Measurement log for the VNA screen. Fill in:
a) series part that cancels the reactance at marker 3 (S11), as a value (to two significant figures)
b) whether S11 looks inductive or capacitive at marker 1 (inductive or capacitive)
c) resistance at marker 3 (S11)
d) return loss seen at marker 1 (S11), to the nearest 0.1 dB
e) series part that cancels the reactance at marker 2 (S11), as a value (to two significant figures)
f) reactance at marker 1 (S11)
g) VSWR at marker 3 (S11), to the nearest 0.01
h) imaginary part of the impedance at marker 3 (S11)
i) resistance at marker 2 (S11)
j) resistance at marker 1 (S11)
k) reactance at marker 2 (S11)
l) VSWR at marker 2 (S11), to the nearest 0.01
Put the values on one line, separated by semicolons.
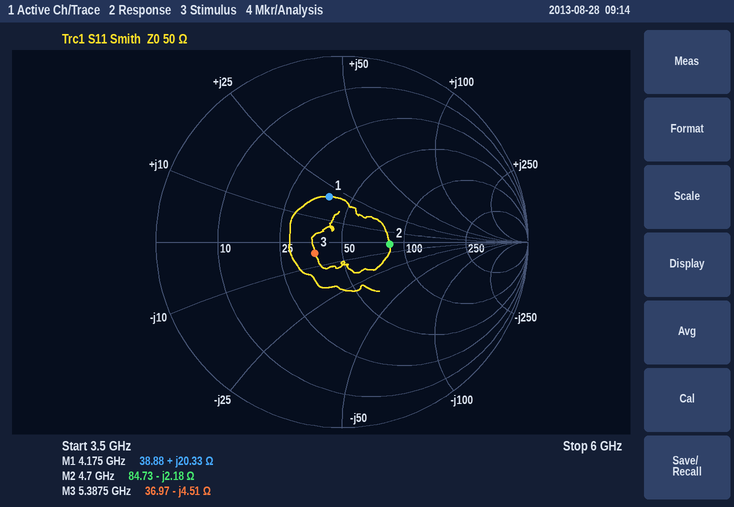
130 pH; inductive; 36.97 Ω; 11.9 dB; 74 pH; +20.33 Ω; 1.38; -4.51 Ω; 84.73 Ω; 38.88 Ω; -2.18 Ω; 1.70
